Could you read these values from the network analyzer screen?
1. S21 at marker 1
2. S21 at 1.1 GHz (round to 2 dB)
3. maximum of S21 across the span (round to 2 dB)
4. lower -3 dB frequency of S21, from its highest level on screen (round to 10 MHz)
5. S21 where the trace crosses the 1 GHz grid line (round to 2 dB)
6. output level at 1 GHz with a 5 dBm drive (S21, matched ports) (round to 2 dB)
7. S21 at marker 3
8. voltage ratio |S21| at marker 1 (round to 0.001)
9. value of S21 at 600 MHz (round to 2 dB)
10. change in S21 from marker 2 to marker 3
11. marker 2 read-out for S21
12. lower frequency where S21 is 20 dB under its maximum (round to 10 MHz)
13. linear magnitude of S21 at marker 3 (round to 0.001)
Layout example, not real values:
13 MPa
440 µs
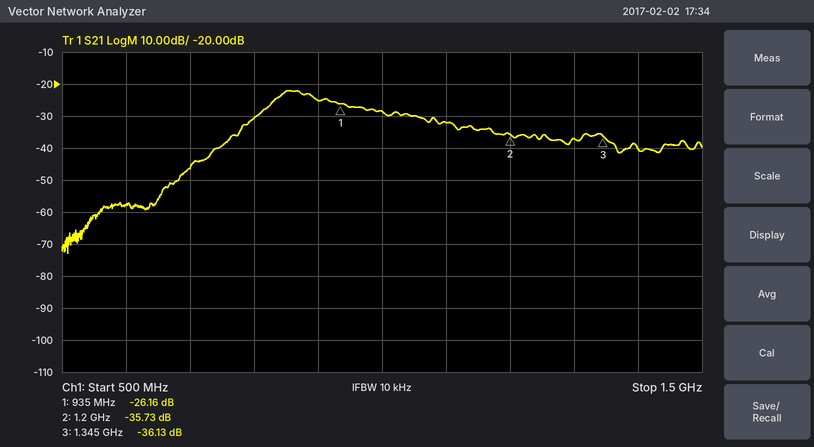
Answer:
-26.16 dB
-32 dB
-22 dB
830 MHz
-28 dB
-24 dBm
-36.13 dB
0.049
-58 dB
-0.40 dB
-35.73 dB
730 MHz
0.016
